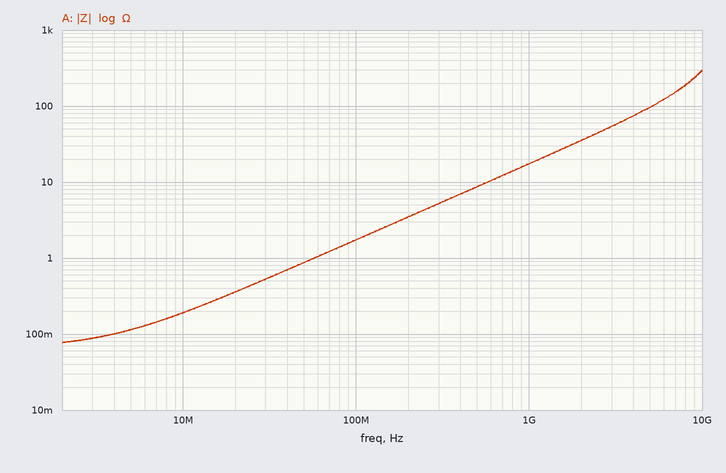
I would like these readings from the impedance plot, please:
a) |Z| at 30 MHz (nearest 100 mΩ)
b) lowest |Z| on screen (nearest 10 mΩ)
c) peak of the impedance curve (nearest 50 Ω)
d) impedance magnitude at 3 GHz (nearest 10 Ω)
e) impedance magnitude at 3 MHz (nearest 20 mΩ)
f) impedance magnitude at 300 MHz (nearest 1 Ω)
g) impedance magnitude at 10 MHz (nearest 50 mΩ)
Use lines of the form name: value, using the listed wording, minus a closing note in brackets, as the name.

|Z| at 30 MHz: 500 mΩ
lowest |Z| on screen: 80 mΩ
peak of the impedance curve: 300 Ω
impedance magnitude at 3 GHz: 50 Ω
impedance magnitude at 3 MHz: 80 mΩ
impedance magnitude at 300 MHz: 5 Ω
impedance magnitude at 10 MHz: 200 mΩ
